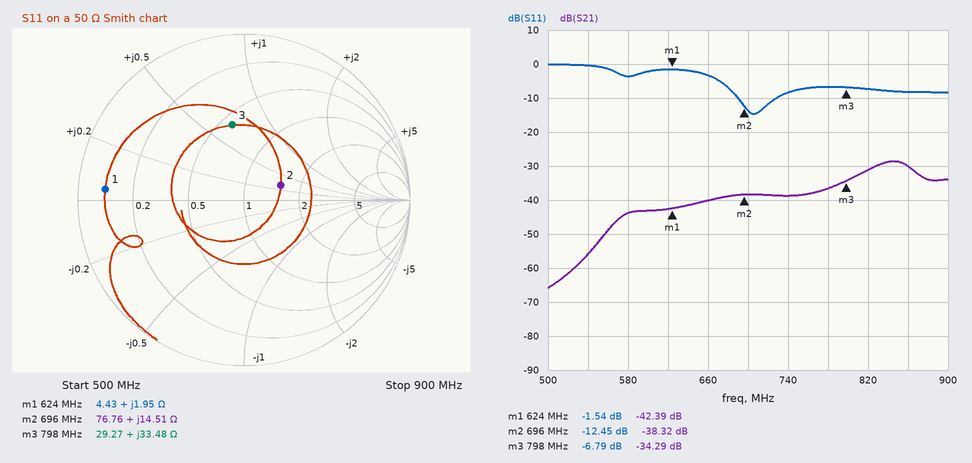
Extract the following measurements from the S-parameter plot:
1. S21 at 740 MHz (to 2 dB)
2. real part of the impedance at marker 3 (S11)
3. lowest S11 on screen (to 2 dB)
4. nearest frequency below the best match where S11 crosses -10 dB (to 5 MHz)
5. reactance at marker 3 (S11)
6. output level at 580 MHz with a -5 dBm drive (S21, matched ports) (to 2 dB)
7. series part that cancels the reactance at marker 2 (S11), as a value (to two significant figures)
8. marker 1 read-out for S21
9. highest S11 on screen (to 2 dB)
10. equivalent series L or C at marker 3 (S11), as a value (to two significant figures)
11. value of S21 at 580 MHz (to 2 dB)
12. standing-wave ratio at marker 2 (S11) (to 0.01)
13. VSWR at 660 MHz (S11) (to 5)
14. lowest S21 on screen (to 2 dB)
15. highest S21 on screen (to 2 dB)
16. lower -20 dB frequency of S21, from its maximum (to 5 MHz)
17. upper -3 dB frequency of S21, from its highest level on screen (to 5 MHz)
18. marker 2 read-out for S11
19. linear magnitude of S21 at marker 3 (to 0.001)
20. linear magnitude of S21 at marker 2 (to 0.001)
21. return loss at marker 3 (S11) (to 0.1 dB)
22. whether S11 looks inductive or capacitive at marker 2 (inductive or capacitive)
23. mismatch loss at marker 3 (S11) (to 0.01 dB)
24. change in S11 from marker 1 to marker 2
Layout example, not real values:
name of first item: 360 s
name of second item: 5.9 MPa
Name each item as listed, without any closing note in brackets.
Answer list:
S21 at 740 MHz: -38 dB
real part of the impedance at marker 3: 29.27 Ω
lowest S11 on screen: -14 dB
nearest frequency below the best match where S11 crosses -10 dB: 690 MHz
reactance at marker 3: +33.48 Ω
output level at 580 MHz with a -5 dBm drive (S21, matched ports): -48 dBm
series part that cancels the reactance at marker 2 (S11), as a value: 16 pF
marker 1 read-out for S21: -42.39 dB
highest S11 on screen: 0 dB
equivalent series L or C at marker 3 (S11), as a value: 6.7 nH
value of S21 at 580 MHz: -44 dB
standing-wave ratio at marker 2 (S11): 1.63
VSWR at 660 MHz (S11): 5
lowest S21 on screen: -66 dB
highest S21 on screen: -28 dB
lower -20 dB frequency of S21, from its maximum: 560 MHz
upper -3 dB frequency of S21, from its highest level on screen: 865 MHz
marker 2 read-out for S11: -12.45 dB
linear magnitude of S21 at marker 3: 0.019
linear magnitude of S21 at marker 2: 0.012
return loss at marker 3 (S11): 6.8 dB
whether S11 looks inductive or capacitive at marker 2: inductive
mismatch loss at marker 3 (S11): 1.02 dB
change in S11 from marker 1 to marker 2: -10.91 dB
